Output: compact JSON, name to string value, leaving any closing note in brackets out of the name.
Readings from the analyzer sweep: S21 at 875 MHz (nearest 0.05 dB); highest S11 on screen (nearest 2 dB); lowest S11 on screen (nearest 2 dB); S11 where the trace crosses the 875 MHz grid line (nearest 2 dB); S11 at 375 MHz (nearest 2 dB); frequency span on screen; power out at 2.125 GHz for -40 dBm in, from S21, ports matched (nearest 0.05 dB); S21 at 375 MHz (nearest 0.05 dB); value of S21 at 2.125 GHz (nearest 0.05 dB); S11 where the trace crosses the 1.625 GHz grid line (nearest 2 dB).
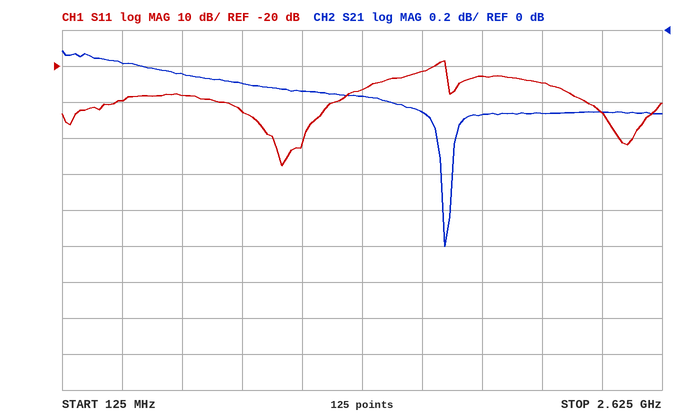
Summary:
{"S21 at 875 MHz": "-0.30 dB", "highest S11 on screen": "-18 dB", "lowest S11 on screen": "-48 dB", "S11 where the trace crosses the 875 MHz grid line": "-32 dB", "S11 at 375 MHz": "-30 dB", "frequency span on screen": "2.5 GHz", "power out at 2.125 GHz for -40 dBm in, from S21, ports matched": "-40.45 dBm", "S21 at 375 MHz": "-0.20 dB", "value of S21 at 2.125 GHz": "-0.45 dB", "S11 where the trace crosses the 1.625 GHz grid line": "-22 dB"}
